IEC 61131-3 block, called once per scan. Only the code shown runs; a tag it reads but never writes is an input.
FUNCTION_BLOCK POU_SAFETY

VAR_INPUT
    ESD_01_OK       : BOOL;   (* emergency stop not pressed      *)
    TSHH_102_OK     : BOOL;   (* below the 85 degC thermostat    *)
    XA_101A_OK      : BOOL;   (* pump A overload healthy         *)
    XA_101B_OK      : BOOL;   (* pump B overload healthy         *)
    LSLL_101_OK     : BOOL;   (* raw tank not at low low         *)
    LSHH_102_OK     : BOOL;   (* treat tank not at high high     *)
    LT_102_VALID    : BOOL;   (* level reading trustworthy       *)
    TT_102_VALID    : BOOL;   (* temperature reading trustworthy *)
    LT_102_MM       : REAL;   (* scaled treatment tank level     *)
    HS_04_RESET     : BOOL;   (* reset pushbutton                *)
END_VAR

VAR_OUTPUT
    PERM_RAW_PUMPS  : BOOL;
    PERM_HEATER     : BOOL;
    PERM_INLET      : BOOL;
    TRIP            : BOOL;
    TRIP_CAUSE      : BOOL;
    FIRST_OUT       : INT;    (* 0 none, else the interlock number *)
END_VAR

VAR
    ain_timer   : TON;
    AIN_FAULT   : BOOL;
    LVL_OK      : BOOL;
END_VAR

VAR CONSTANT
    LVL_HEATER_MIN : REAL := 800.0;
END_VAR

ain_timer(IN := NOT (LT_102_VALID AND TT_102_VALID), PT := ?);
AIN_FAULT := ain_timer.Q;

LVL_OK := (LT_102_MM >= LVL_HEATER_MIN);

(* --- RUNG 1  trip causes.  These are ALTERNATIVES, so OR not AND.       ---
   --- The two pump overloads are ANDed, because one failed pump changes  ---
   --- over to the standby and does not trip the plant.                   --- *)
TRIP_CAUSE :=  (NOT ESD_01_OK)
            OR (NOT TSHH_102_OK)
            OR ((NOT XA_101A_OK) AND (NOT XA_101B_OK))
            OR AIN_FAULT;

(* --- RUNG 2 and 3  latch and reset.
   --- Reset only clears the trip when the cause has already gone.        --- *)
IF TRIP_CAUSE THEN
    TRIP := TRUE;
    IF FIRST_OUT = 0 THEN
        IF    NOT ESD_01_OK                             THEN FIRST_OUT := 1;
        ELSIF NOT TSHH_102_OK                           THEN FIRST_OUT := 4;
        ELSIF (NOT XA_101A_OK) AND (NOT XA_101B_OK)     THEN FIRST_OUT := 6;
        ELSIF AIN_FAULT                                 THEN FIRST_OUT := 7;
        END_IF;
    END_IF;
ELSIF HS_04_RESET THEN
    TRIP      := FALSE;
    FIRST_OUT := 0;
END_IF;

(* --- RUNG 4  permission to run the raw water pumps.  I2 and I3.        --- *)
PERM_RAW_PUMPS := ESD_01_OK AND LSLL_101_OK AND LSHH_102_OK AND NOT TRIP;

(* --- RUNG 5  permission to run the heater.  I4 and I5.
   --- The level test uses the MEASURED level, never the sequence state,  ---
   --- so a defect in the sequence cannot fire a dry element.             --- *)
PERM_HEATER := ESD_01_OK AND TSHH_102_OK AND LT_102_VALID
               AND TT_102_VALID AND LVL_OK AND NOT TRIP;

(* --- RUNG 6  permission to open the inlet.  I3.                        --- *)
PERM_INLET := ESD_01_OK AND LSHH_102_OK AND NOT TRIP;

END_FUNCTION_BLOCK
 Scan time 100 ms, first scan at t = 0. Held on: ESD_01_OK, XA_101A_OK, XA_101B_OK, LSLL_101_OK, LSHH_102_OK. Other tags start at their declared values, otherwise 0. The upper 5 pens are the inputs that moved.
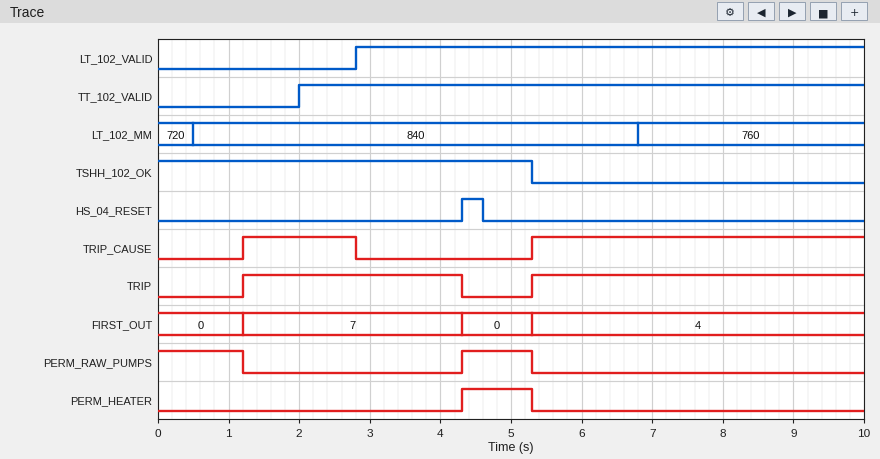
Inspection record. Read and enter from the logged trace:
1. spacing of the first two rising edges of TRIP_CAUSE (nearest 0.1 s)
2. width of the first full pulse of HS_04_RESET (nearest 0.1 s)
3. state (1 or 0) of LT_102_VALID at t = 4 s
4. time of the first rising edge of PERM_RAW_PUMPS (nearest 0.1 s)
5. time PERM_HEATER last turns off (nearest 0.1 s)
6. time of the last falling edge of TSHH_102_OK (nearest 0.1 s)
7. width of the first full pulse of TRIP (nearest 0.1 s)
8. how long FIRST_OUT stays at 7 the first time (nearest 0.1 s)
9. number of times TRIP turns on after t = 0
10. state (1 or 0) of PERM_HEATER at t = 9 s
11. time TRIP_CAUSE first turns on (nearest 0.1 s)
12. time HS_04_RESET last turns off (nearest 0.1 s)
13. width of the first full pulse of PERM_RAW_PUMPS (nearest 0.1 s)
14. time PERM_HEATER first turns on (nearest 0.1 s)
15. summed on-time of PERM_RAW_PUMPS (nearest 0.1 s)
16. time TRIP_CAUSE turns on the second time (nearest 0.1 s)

4.1 s
0.3 s
1
4.3 s
5.3 s
5.3 s
3.1 s
3.1 s
2
0
1.2 s
4.6 s
1.0 s
4.3 s
2.2 s
5.3 s
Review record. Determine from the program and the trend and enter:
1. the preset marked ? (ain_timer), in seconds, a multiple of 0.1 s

1.2 s
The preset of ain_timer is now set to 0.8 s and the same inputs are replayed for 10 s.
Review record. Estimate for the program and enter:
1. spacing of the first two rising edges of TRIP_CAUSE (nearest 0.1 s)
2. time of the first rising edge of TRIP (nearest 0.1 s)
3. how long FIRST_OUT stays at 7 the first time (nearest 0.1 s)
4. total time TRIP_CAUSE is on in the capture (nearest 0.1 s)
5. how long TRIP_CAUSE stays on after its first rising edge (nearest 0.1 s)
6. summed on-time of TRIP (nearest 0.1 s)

4.5 s
0.8 s
3.5 s
6.7 s
2.0 s
8.2 s
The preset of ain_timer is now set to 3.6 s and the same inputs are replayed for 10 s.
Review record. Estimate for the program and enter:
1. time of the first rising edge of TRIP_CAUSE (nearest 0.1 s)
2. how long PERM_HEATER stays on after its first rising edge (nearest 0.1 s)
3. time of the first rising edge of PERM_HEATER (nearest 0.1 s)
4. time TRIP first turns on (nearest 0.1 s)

5.3 s
2.5 s
2.8 s
5.3 s
